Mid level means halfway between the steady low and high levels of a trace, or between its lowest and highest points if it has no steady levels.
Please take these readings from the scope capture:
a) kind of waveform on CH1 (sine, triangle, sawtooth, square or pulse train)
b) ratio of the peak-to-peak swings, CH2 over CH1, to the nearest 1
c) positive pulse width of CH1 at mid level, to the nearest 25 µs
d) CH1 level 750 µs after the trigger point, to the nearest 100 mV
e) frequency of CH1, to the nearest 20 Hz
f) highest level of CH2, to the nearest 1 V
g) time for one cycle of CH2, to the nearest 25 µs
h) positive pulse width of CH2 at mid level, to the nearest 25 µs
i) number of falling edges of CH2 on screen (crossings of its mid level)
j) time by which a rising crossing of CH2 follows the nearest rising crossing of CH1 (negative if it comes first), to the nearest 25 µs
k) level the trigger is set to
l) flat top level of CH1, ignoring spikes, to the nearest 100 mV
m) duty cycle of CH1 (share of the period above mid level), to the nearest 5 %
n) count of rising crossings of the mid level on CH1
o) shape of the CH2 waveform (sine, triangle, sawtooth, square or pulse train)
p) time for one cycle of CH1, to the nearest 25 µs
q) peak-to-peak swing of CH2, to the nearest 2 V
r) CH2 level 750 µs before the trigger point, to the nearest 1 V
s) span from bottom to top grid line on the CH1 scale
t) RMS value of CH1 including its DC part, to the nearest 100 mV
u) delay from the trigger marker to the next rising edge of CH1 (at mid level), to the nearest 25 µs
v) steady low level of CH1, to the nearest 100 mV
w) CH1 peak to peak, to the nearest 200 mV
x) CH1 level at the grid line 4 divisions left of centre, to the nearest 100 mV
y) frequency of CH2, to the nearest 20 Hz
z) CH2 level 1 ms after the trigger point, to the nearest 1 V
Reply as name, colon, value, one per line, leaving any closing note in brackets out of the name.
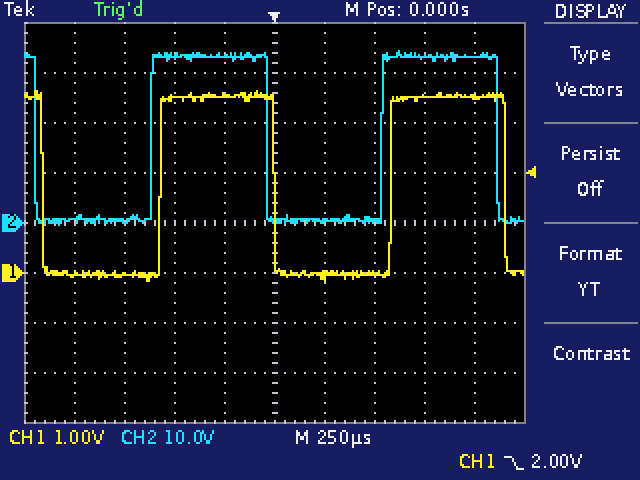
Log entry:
kind of waveform on CH1: square
ratio of the peak-to-peak swings, CH2 over CH1, to the nearest 1: 9
positive pulse width of CH1 at mid level, to the nearest 25 µs: 575 µs
CH1 level 750 µs after the trigger point, to the nearest 100 mV: 3.5 V
frequency of CH1, to the nearest 20 Hz: 860 Hz
highest level of CH2, to the nearest 1 V: 34 V
time for one cycle of CH2, to the nearest 25 µs: 1.150 ms
positive pulse width of CH2 at mid level, to the nearest 25 µs: 575 µs
number of falling edges of CH2 on screen: 3
time by which a rising crossing of CH2 follows the nearest rising crossing of CH1 (negative if it comes first), to the nearest 25 µs: -50 µs
level the trigger is set to: 2.00 V
flat top level of CH1, ignoring spikes, to the nearest 100 mV: 3.5 V
duty cycle of CH1 (share of the period above mid level), to the nearest 5 %: 50 %
count of rising crossings of the mid level on CH1: 2
shape of the CH2 waveform: square
time for one cycle of CH1, to the nearest 25 µs: 1.150 ms
peak-to-peak swing of CH2, to the nearest 2 V: 34 V
CH2 level 750 µs before the trigger point, to the nearest 1 V: 0 V
span from bottom to top grid line on the CH1 scale: 8 V
RMS value of CH1 including its DC part, to the nearest 100 mV: 2.5 V
delay from the trigger marker to the next rising edge of CH1 (at mid level), to the nearest 25 µs: 575 µs
steady low level of CH1, to the nearest 100 mV: 0.0 V
CH1 peak to peak, to the nearest 200 mV: 3.8 V
CH1 level at the grid line 4 divisions left of centre, to the nearest 100 mV: 0.0 V
frequency of CH2, to the nearest 20 Hz: 860 Hz
CH2 level 1 ms after the trigger point, to the nearest 1 V: 33 V
